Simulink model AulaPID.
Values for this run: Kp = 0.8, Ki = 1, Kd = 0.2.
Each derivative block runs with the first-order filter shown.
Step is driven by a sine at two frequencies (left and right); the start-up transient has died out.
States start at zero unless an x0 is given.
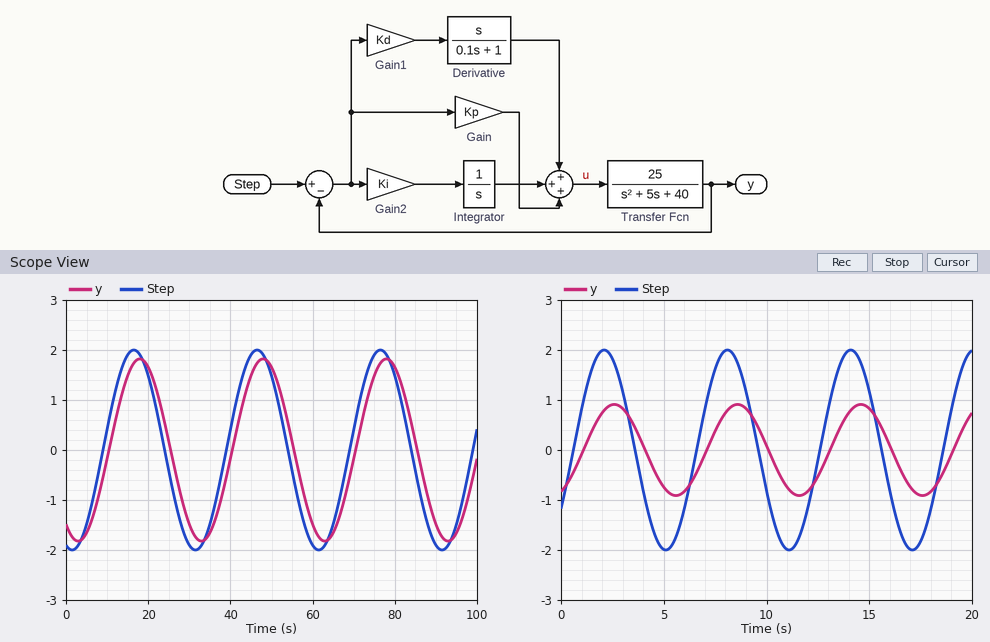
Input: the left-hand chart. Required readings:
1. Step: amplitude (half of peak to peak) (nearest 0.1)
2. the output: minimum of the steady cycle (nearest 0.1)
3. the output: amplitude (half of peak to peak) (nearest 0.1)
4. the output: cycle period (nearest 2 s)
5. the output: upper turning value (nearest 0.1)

2.0
-1.8
1.8
30 s
1.8
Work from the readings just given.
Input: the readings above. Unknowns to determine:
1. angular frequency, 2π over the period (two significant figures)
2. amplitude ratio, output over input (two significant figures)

0.21 rad/s
0.90
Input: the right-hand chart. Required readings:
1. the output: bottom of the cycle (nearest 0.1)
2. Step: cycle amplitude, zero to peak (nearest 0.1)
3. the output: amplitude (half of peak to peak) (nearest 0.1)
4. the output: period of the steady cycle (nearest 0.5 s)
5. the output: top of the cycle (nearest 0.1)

-0.9
2.0
0.9
6.0 s
0.9
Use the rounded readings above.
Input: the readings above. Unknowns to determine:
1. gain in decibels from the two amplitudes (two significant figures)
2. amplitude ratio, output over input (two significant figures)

-6.9 dB
0.45
